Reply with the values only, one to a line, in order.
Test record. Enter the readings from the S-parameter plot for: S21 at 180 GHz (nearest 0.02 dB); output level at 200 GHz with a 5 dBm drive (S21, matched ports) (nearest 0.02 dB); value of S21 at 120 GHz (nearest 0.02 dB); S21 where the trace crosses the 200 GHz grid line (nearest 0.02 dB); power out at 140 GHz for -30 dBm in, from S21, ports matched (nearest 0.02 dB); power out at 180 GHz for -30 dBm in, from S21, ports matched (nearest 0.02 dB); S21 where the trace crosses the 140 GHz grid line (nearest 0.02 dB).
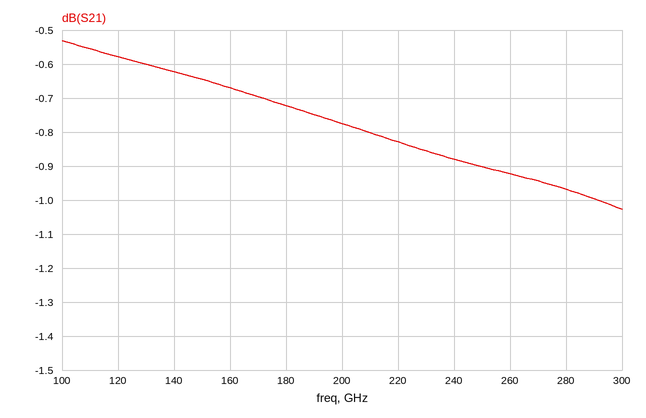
-0.72 dB
4.22 dBm
-0.58 dB
-0.78 dB
-30.62 dBm
-30.72 dBm
-0.62 dB
